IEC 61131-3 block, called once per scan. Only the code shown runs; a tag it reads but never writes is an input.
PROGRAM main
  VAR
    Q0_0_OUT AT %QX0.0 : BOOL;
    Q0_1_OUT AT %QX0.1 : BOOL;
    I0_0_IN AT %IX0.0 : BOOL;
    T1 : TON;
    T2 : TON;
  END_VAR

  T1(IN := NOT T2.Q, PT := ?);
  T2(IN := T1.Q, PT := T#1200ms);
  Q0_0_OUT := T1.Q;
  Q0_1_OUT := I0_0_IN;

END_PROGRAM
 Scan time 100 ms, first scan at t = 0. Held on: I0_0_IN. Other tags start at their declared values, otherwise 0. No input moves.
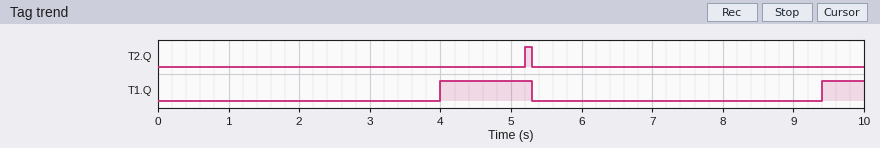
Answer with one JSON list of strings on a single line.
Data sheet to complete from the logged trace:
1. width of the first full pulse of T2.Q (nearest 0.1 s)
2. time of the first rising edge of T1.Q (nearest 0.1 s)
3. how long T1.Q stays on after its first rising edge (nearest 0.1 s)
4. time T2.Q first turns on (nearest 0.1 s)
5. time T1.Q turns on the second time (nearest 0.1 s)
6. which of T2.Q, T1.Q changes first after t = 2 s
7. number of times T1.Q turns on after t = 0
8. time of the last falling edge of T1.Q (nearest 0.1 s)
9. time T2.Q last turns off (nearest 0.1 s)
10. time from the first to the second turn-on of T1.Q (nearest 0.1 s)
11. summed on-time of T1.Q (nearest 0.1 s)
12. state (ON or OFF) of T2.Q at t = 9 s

["0.1 s", "4.0 s", "1.3 s", "5.2 s", "9.4 s", "T1.Q", "2", "5.3 s", "5.3 s", "5.4 s", "1.9 s", "OFF"]
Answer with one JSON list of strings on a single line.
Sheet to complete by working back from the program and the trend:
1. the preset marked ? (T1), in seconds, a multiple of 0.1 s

["4.0 s"]
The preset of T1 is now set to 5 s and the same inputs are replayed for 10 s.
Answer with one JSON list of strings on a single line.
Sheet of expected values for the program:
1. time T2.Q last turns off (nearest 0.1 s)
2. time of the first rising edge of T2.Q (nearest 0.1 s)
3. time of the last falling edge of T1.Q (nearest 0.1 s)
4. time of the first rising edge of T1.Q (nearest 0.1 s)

["6.3 s", "6.2 s", "6.3 s", "5.0 s"]
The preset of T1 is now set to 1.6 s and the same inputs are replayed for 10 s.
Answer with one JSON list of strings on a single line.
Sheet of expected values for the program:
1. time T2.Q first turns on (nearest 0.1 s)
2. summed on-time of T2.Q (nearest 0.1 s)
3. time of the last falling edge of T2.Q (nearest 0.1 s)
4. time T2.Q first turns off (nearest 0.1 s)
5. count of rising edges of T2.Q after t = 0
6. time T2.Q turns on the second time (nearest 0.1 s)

["2.8 s", "0.3 s", "8.9 s", "2.9 s", "3", "5.8 s"]
